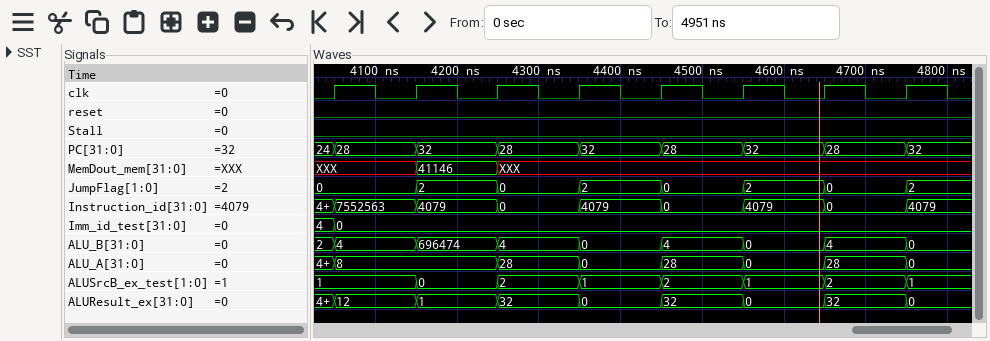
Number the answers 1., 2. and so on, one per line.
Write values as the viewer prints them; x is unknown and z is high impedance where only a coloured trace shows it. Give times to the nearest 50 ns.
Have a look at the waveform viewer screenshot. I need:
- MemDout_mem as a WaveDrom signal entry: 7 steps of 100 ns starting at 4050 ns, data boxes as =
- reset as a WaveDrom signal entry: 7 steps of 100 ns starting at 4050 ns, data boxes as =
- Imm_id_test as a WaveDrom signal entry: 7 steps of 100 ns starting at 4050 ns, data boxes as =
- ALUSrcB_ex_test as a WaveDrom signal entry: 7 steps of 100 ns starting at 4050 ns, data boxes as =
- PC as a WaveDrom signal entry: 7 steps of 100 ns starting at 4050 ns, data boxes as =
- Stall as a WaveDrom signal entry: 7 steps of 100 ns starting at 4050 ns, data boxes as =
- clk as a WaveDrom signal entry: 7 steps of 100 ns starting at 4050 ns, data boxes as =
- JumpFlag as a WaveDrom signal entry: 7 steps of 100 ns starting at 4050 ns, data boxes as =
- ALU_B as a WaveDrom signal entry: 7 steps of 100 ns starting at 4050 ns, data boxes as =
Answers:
1. {name: 'MemDout_mem', wave: 'x=x....', data: '41146'}
2. {name: 'reset', wave: '0......'}
3. {name: 'Imm_id_test', wave: '=......', data: '0'}
4. {name: 'ALUSrcB_ex_test', wave: '=======', data: '1 0 2 1 2 1 2'}
5. {name: 'PC', wave: '=======', data: '28 32 28 32 28 32 28'}
6. {name: 'Stall', wave: '0......'}
7. {name: 'clk', wave: 'p......'}
8. {name: 'JumpFlag', wave: '=======', data: '0 2 0 2 0 2 0'}
9. {name: 'ALU_B', wave: '=======', data: '4 696474 4 0 4 0 4'}
